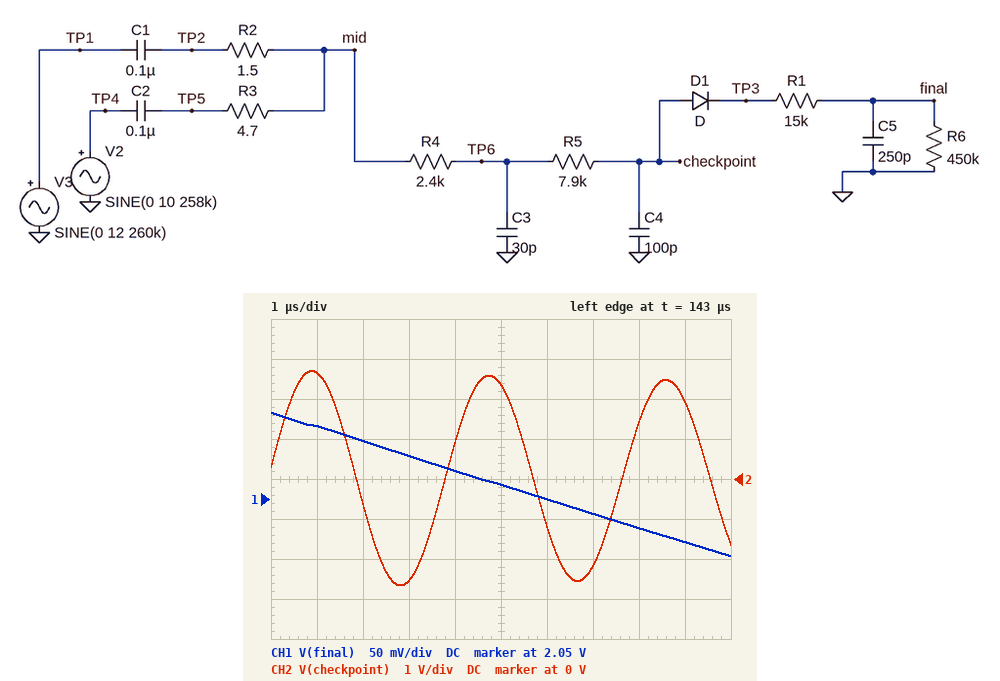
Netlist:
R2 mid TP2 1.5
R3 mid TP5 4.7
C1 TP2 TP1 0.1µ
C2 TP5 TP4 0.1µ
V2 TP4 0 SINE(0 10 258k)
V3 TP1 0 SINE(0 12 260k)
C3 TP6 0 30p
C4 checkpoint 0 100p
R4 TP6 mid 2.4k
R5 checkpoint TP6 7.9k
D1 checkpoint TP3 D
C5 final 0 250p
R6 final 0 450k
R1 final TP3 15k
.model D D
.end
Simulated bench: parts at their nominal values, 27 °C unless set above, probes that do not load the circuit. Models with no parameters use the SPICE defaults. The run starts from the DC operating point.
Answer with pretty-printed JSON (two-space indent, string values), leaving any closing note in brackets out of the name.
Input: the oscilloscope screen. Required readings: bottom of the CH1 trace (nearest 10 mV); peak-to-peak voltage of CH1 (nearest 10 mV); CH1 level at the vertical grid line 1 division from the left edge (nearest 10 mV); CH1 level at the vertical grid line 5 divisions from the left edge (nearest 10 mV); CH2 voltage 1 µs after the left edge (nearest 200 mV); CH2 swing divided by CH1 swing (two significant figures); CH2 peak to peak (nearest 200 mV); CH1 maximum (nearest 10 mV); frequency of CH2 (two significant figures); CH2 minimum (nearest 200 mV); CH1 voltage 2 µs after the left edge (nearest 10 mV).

{
  "bottom of the CH1 trace": "1.98 V",
  "peak-to-peak voltage of CH1": "180 mV",
  "CH1 level at the vertical grid line 1 division from the left edge": "2.14 V",
  "CH1 level at the vertical grid line 5 divisions from the left edge": "2.07 V",
  "CH2 voltage 1 µs after the left edge": "2.6 V",
  "CH2 swing divided by CH1 swing": "30",
  "CH2 peak to peak": "5.4 V",
  "CH1 maximum": "2.16 V",
  "frequency of CH2": "260 kHz",
  "CH2 minimum": "-2.6 V",
  "CH1 voltage 2 µs after the left edge": "2.12 V"
}
